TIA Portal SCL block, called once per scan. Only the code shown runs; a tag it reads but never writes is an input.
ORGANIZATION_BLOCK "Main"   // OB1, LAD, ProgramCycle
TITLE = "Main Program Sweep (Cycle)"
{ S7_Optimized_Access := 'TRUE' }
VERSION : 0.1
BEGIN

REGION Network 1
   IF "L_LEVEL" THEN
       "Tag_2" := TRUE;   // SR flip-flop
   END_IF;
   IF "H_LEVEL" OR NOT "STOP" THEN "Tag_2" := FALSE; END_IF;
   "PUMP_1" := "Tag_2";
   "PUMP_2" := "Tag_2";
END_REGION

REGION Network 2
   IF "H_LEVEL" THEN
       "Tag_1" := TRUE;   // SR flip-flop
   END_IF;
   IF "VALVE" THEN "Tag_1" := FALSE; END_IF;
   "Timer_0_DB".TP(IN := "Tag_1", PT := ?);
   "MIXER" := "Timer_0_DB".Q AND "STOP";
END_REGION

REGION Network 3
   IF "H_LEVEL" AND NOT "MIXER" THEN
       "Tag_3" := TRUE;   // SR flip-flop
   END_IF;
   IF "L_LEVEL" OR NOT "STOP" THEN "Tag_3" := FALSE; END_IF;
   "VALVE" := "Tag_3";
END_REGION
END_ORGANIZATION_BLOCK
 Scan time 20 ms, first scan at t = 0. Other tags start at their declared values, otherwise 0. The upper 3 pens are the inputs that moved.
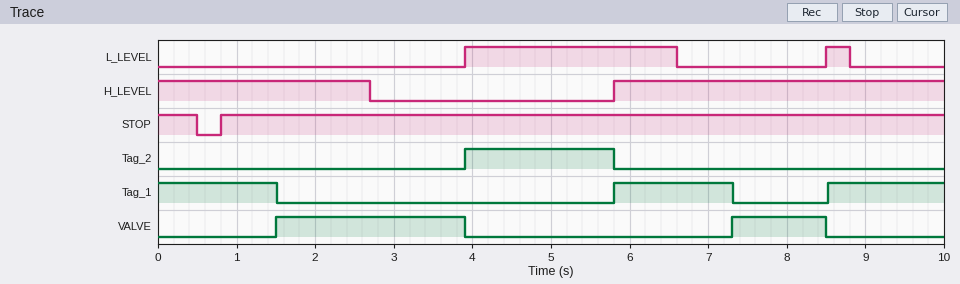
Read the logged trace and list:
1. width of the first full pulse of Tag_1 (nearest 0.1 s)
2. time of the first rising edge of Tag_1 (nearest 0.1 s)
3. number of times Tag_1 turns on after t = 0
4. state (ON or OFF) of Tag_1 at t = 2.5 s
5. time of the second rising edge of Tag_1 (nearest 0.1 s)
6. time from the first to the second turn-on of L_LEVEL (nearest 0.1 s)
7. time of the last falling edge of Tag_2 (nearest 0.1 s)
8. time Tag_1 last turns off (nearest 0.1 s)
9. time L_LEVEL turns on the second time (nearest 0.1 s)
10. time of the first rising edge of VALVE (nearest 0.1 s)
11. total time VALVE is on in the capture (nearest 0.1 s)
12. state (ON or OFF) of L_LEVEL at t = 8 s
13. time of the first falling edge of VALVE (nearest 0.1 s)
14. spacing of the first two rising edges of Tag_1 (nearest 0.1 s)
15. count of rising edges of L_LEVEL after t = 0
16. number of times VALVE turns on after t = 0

1.5 s
5.8 s
2
OFF
8.5 s
4.6 s
5.8 s
7.3 s
8.5 s
1.5 s
3.6 s
OFF
3.9 s
2.7 s
2
2
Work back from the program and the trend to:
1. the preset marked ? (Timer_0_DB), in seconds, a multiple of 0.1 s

1.5 s
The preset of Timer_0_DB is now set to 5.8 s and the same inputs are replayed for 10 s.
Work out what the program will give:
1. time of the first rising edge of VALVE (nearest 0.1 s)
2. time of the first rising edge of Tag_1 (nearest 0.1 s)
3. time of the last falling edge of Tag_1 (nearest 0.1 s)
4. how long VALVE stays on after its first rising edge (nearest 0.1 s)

6.6 s
8.5 s
6.6 s
1.9 s
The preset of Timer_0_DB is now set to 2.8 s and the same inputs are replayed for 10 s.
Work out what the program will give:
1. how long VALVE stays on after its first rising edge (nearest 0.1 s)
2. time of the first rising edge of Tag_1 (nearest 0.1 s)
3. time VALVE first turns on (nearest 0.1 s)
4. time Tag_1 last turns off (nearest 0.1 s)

1.9 s
8.5 s
6.6 s
6.6 s
